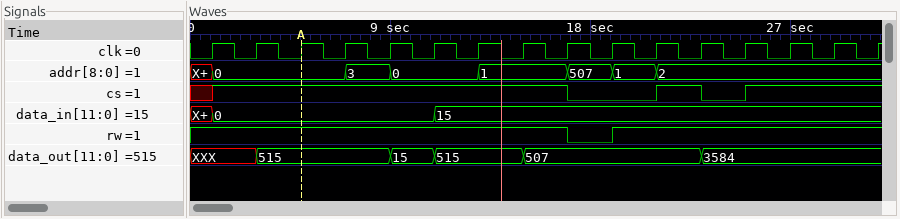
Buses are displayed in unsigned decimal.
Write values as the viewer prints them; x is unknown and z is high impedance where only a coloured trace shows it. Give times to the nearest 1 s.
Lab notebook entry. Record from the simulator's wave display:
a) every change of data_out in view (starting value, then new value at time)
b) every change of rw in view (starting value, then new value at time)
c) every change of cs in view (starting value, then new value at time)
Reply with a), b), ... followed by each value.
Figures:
a) XXX, 515 at 3 s, 15 at 9 s, 515 at 11 s, 507 at 15 s, 3584 at 23 s
b) 1, 0 at 17 s, 1 at 19 s
c) x, 1 at 1 s, 0 at 17 s, 1 at 21 s, 0 at 23 s, 1 at 25 s
